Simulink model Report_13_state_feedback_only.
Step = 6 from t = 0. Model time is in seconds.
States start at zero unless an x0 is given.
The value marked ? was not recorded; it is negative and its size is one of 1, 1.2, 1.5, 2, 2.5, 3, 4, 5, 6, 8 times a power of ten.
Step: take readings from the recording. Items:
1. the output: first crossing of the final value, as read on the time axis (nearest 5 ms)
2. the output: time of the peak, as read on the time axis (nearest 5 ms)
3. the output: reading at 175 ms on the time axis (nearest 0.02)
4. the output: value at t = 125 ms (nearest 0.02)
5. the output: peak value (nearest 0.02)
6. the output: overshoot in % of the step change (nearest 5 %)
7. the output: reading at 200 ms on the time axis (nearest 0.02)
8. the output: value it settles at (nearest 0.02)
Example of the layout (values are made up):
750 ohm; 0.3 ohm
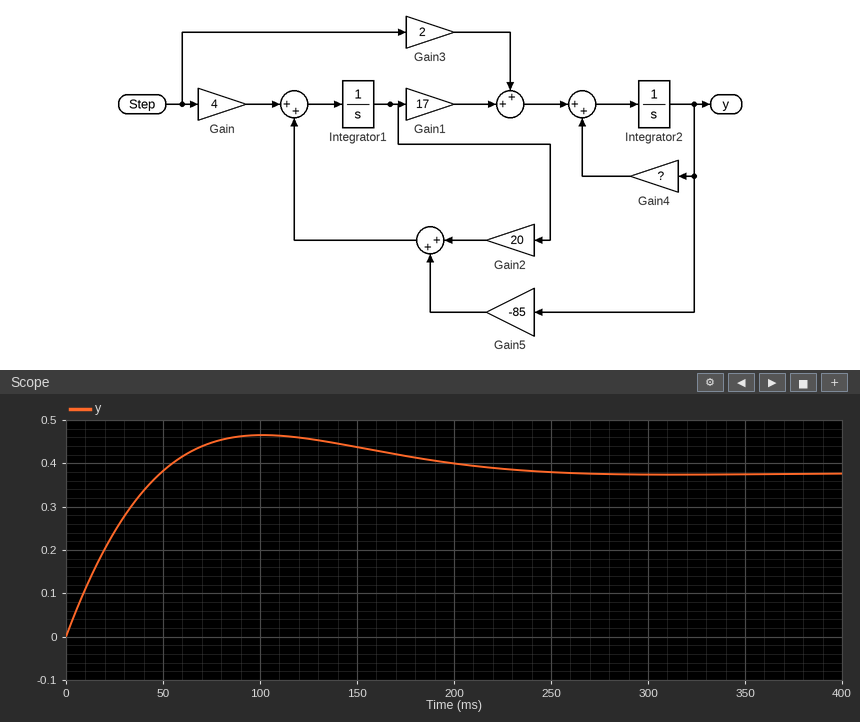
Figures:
50 ms; 100 ms; 0.42; 0.46; 0.46; 25 %; 0.40; 0.38
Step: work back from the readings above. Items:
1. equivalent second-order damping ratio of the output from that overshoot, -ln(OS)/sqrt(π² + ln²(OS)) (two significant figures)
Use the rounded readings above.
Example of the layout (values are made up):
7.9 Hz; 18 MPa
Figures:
0.40
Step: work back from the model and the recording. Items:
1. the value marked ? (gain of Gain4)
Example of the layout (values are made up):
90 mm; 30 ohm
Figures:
-50
